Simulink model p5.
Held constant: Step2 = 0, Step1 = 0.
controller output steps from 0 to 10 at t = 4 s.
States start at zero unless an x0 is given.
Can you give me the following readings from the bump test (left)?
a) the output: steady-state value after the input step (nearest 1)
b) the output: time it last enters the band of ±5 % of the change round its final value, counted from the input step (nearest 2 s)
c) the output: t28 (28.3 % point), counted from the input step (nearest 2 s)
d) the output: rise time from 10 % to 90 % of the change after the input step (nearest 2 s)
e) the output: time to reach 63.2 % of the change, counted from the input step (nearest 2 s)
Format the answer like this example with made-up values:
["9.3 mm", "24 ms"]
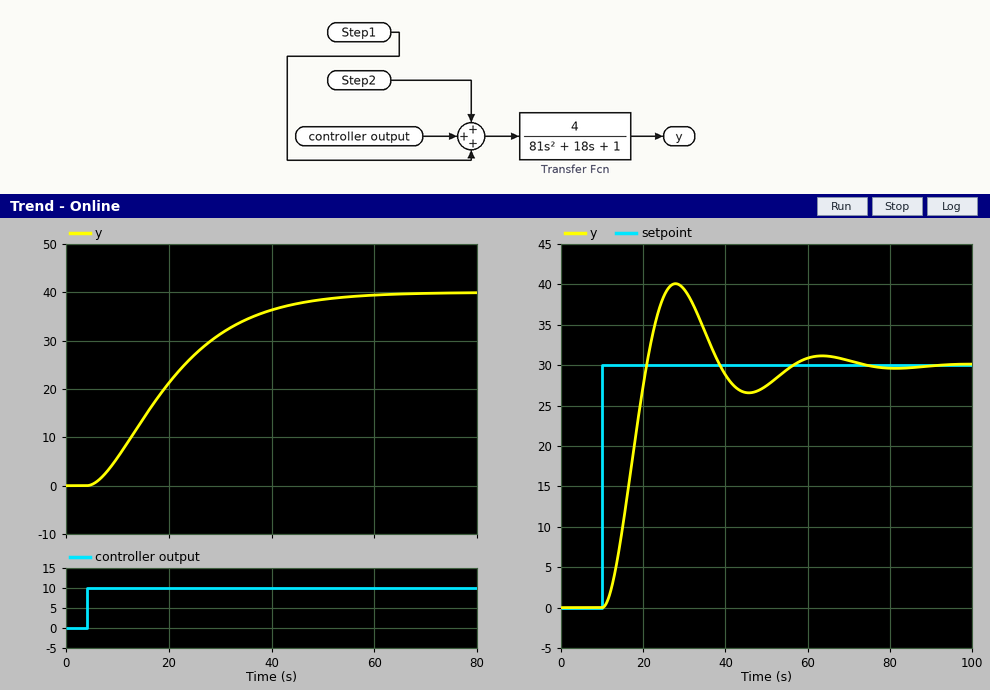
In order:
["40", "42 s", "10 s", "30 s", "20 s"]
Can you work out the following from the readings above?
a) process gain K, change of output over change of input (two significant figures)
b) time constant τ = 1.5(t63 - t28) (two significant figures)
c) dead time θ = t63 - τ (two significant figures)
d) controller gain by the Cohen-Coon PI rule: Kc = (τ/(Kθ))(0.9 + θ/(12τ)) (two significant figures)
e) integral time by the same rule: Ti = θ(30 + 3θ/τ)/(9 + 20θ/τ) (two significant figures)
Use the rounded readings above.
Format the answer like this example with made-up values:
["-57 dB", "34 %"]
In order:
["4.0", "15 s", "5.0 s", "0.70", "9.9 s"]
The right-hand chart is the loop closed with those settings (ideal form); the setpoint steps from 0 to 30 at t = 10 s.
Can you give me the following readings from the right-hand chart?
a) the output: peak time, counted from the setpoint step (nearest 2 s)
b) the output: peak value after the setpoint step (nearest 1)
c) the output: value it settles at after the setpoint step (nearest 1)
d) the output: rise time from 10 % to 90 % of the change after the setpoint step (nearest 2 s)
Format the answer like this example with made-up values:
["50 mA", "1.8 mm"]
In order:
["18 s", "40", "30", "8 s"]
